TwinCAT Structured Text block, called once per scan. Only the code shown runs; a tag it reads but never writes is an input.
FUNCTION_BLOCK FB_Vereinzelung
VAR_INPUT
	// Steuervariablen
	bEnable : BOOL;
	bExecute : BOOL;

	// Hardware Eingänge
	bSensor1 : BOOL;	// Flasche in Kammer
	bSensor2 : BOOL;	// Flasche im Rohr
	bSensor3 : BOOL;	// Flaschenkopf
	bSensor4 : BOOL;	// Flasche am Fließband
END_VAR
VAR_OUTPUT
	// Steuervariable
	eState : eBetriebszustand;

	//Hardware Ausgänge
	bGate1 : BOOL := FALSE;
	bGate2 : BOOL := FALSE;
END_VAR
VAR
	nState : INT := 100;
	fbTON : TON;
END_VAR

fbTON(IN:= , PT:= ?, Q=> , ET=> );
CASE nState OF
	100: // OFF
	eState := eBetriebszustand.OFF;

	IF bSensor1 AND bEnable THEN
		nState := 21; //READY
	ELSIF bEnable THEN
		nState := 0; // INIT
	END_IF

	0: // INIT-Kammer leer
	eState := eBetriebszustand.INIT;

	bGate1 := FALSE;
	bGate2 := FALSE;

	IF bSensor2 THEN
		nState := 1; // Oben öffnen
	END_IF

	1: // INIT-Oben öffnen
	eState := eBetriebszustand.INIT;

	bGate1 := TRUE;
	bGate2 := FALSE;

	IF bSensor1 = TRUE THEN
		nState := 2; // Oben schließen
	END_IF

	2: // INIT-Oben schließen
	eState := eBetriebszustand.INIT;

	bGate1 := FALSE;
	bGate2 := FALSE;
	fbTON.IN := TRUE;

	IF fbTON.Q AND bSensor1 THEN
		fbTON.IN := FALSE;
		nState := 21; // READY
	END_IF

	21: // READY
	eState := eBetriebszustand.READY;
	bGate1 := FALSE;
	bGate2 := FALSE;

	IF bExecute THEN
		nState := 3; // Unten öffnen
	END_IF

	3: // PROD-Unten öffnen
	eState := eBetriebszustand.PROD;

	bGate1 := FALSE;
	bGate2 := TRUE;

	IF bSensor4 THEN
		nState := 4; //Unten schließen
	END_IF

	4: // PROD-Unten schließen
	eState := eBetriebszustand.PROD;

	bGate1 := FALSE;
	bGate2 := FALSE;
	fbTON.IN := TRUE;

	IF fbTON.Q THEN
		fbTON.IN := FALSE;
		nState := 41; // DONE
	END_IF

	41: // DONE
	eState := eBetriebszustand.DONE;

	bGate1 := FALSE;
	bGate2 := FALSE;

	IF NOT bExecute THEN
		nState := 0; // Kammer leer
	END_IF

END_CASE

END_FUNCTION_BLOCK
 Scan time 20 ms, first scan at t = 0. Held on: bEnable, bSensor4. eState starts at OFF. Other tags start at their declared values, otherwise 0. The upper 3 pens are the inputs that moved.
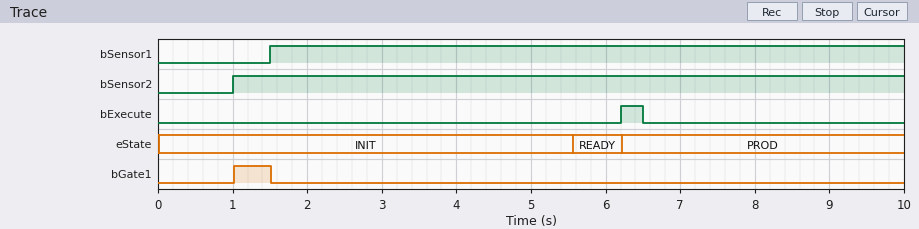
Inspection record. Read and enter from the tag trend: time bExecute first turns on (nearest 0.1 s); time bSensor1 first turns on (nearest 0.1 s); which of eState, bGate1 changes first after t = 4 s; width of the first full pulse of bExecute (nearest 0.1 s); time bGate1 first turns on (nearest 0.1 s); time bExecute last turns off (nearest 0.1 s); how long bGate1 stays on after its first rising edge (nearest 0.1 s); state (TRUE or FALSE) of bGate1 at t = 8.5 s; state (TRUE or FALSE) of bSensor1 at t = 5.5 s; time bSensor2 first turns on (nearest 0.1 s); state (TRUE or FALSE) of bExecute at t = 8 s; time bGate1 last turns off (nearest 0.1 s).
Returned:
6.2 s
1.5 s
eState
0.3 s
1.0 s
6.5 s
0.5 s
FALSE
TRUE
1.0 s
FALSE
1.5 s
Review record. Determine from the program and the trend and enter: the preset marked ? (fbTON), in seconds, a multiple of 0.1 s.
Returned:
4.0 s
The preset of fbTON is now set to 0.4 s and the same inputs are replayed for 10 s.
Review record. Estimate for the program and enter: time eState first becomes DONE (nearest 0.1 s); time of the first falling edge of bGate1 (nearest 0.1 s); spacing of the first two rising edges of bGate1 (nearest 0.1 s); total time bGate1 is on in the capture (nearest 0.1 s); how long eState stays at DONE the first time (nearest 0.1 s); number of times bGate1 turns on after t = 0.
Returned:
6.7 s
1.5 s
5.7 s
0.5 s
0.0 s
2
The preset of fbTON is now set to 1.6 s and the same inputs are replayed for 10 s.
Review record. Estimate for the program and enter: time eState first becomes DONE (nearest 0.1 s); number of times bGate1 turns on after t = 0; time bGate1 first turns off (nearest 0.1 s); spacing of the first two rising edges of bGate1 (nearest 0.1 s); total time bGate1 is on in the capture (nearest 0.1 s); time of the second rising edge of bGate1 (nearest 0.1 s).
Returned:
7.9 s
2
1.5 s
6.9 s
0.5 s
7.9 s
